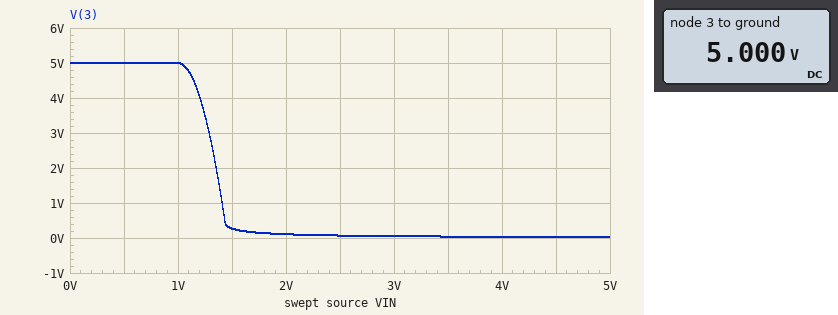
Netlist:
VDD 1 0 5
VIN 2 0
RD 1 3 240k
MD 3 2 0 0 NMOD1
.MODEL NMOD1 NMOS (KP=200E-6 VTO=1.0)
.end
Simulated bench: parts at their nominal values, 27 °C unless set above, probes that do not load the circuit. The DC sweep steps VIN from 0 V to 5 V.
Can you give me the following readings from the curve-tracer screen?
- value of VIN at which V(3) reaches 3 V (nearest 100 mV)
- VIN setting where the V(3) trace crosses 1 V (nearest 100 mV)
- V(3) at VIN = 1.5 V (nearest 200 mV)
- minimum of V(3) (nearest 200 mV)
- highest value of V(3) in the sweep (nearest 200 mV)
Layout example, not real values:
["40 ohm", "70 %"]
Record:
["1.3 V", "1.4 V", "200 mV", "0 V", "5.0 V"]
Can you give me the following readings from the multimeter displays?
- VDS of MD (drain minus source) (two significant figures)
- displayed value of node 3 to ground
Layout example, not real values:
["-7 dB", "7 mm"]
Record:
["5.0 V", "5.000 V"]
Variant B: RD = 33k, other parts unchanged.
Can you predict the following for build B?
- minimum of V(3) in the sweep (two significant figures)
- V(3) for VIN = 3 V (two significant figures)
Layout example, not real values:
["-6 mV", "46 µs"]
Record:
["190 mV", "390 mV"]
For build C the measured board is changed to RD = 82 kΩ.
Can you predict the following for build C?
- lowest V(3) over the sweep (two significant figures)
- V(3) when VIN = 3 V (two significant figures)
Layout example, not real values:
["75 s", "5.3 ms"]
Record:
["76 mV", "150 mV"]
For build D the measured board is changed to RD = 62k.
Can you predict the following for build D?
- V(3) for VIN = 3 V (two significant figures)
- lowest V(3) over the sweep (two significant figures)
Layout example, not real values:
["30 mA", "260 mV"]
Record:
["200 mV", "100 mV"]
